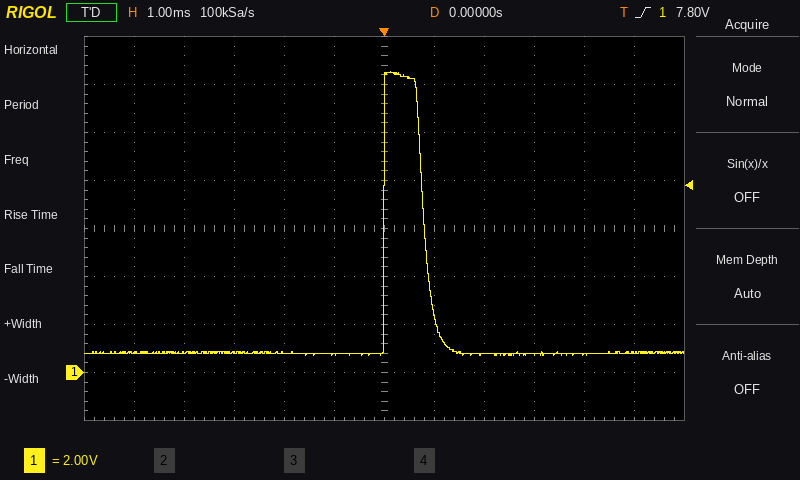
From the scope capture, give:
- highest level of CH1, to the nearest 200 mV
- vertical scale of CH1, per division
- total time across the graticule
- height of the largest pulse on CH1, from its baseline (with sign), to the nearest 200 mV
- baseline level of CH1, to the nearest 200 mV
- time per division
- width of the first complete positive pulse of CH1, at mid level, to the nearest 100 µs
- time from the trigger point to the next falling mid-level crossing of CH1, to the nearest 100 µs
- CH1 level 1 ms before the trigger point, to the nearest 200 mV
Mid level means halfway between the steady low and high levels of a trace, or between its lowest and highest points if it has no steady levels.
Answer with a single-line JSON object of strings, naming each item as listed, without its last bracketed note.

{"highest level of CH1, to the nearest 200 mV": "12.6 V", "vertical scale of CH1, per division": "2 V", "total time across the graticule": "12 ms", "height of the largest pulse on CH1, from its baseline (with sign), to the nearest 200 mV": "+11.8 V", "baseline level of CH1, to the nearest 200 mV": "800 mV", "time per division": "1 ms", "width of the first complete positive pulse of CH1, at mid level, to the nearest 100 µs": "800 µs", "time from the trigger point to the next falling mid-level crossing of CH1, to the nearest 100 µs": "800 µs", "CH1 level 1 ms before the trigger point, to the nearest 200 mV": "800 mV"}
